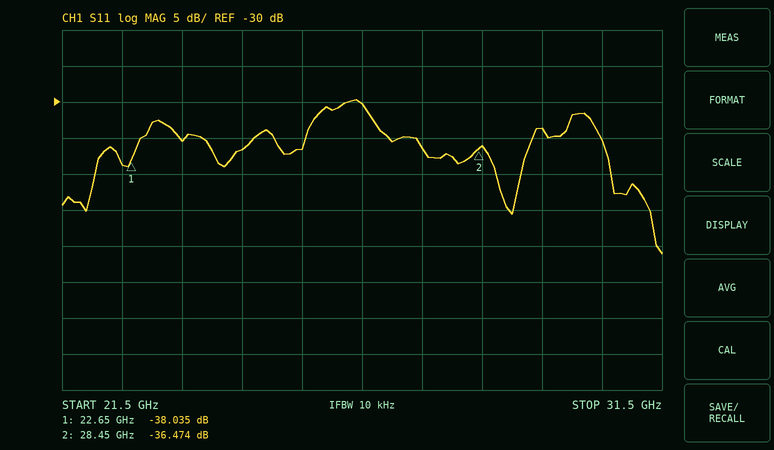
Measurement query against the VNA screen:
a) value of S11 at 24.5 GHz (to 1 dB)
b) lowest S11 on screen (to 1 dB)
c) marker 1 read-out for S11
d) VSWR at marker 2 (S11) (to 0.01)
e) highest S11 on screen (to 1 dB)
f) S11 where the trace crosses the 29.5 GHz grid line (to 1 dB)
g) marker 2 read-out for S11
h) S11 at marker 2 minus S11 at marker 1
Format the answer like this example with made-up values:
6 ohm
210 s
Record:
-37 dB
-51 dB
-38.035 dB
1.03
-30 dB
-34 dB
-36.474 dB
1.561 dB
